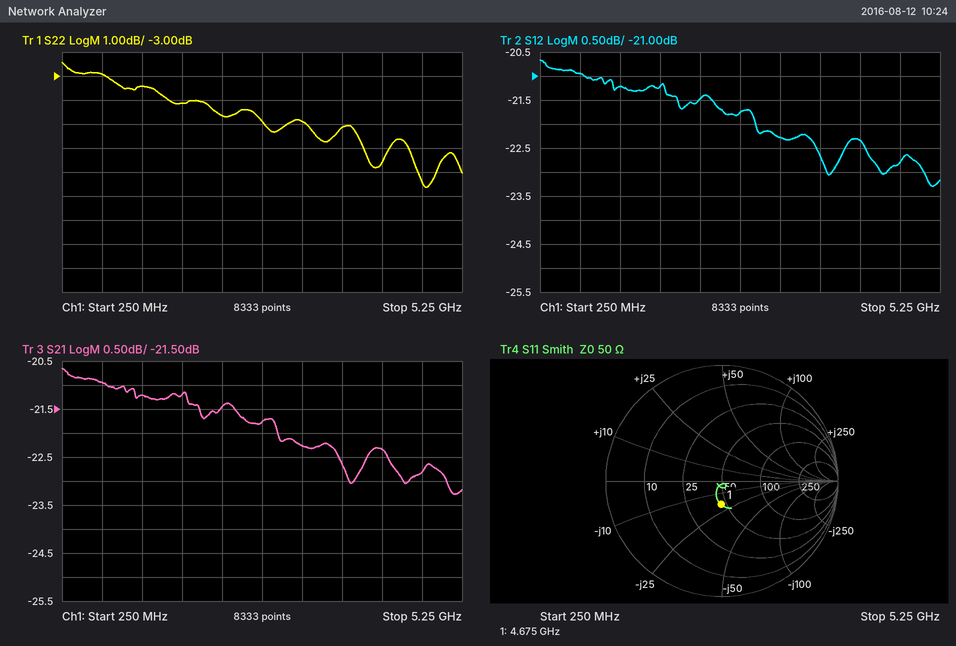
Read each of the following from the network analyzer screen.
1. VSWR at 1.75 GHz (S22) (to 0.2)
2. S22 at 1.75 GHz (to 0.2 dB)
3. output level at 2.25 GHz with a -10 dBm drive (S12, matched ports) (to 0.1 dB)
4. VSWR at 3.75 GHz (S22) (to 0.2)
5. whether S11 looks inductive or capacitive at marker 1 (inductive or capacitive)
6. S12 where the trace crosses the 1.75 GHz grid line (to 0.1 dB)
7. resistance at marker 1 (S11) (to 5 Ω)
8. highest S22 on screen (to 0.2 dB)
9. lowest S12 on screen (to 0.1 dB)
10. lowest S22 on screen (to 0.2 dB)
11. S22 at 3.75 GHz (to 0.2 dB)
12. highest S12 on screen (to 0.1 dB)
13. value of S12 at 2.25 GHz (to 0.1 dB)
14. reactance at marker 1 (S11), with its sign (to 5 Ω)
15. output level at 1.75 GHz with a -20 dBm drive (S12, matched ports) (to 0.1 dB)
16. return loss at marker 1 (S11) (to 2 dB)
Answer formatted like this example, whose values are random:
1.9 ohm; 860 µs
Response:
4.2; -4.2 dB; -31.5 dBm; 3.4; capacitive; -21.2 dB; 45 Ω; -2.4 dB; -23.3 dB; -7.6 dB; -5.2 dB; -20.7 dB; -21.5 dB; -20 Ω; -41.2 dBm; 14 dB
